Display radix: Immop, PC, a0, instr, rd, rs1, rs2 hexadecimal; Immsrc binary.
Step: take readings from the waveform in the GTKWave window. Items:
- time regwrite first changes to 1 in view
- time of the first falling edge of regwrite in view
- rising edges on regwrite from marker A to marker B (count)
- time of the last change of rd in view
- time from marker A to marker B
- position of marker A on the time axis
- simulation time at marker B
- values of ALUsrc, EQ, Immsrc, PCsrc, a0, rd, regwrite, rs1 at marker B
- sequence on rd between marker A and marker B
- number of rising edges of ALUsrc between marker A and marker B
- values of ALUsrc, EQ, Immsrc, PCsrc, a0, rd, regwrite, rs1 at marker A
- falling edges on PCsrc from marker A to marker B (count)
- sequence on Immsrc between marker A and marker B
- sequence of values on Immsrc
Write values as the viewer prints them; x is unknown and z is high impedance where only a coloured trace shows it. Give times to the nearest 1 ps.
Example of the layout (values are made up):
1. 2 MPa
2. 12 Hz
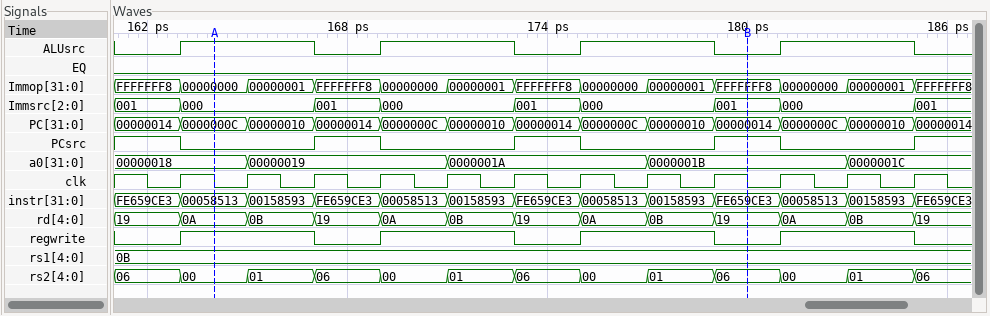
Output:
1. 163 ps
2. 167 ps
3. 2
4. 185 ps
5. 16 ps
6. 164 ps
7. 180 ps
8. ALUsrc=0, EQ=0, Immsrc=001, PCsrc=1, a0=0000001B, rd=19, regwrite=0, rs1=0B
9. 0A, 0B, 19, 0A, 0B, 19, 0A, 0B, 19
10. 2
11. ALUsrc=1, EQ=0, Immsrc=000, PCsrc=0, a0=00000018, rd=0A, regwrite=1, rs1=0B
12. 2
13. 000, 001, 000, 001, 000, 001
14. 001, 000, 001, 000, 001, 000, 001, 000, 001
